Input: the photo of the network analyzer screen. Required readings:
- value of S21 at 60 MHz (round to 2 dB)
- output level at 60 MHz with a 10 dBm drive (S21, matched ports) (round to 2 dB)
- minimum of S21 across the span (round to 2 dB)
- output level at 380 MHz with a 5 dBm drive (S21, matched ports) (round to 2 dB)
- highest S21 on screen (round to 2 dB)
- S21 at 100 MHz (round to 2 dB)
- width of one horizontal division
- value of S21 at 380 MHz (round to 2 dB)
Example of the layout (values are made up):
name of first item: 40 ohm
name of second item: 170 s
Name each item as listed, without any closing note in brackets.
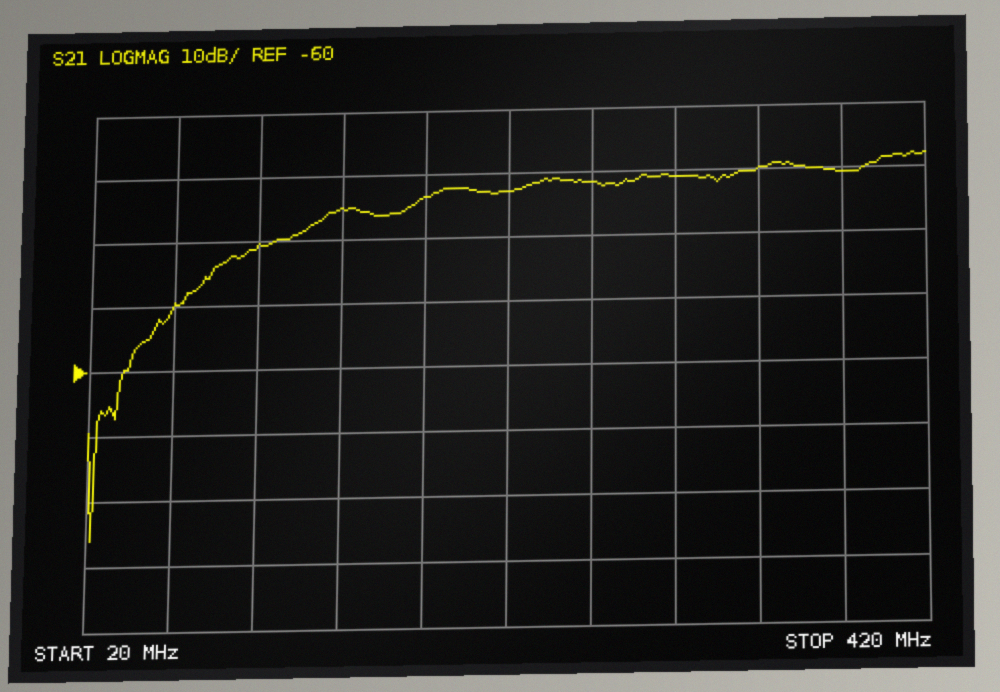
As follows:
value of S21 at 60 MHz: -50 dB
output level at 60 MHz with a 10 dBm drive (S21, matched ports): -40 dBm
minimum of S21 across the span: -86 dB
output level at 380 MHz with a 5 dBm drive (S21, matched ports): -26 dBm
highest S21 on screen: -28 dB
S21 at 100 MHz: -40 dB
width of one horizontal division: 40 MHz
value of S21 at 380 MHz: -30 dB
